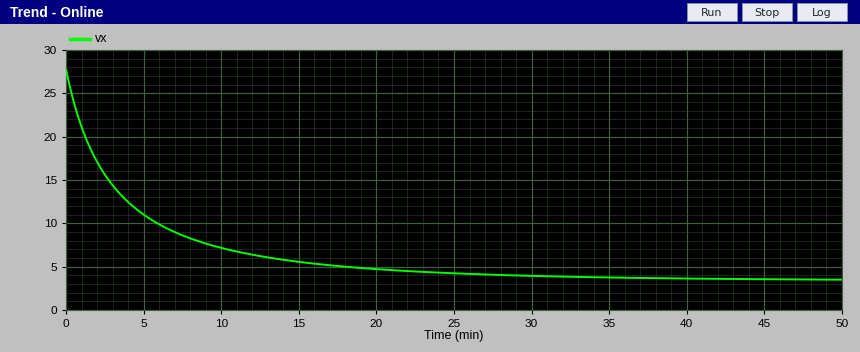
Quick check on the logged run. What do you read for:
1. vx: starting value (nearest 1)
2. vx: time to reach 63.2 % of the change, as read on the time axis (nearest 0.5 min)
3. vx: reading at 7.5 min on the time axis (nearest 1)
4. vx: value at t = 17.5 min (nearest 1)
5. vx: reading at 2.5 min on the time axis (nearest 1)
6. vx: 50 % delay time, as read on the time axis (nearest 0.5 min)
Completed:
28
4.0 min
9
5
16
2.5 min
